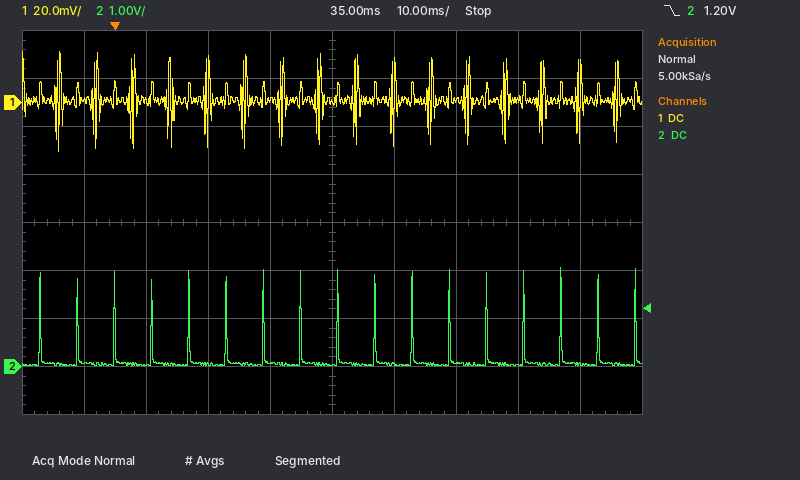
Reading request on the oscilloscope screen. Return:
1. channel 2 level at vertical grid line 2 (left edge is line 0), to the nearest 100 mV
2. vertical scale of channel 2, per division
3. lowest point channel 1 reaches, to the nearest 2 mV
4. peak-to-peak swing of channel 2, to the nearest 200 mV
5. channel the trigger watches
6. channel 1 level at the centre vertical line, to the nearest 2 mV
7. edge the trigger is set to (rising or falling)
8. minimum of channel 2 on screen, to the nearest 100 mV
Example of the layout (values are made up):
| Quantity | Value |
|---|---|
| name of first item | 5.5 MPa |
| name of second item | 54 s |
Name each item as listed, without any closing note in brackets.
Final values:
| Quantity | Value |
|---|---|
| channel 2 level at vertical grid line 2 (left edge is line 0), to the nearest 100 mV | 0.0 V |
| vertical scale of channel 2, per division | 1 V |
| lowest point channel 1 reaches, to the nearest 2 mV | -20 mV |
| peak-to-peak swing of channel 2, to the nearest 200 mV | 2.0 V |
| channel the trigger watches | channel 2 |
| channel 1 level at the centre vertical line, to the nearest 2 mV | 0 mV |
| edge the trigger is set to | falling |
| minimum of channel 2 on screen, to the nearest 100 mV | 0.0 V |
